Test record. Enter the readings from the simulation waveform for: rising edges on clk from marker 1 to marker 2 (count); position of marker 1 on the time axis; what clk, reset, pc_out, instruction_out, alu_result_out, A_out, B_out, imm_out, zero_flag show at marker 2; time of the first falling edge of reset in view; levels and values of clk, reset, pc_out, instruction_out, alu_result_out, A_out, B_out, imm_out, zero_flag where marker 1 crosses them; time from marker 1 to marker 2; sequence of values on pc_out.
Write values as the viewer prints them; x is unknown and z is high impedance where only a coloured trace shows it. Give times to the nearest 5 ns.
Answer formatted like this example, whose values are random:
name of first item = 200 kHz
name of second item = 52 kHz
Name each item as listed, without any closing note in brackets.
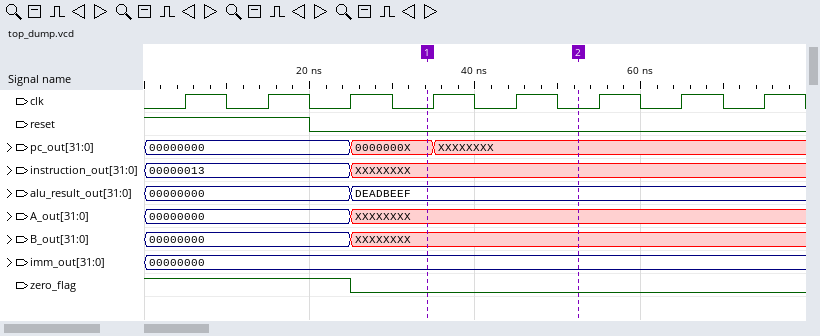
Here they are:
rising edges on clk from marker 1 to marker 2 = 2
position of marker 1 on the time axis = 35 ns
what clk, reset, pc_out, instruction_out, alu_result_out, A_out, B_out, imm_out, zero_flag show at marker 2 = clk=0, reset=0, pc_out=XXXXXXXX, instruction_out=XXXXXXXX, alu_result_out=DEADBEEF, A_out=XXXXXXXX, B_out=XXXXXXXX, imm_out=00000000, zero_flag=0
time of the first falling edge of reset in view = 20 ns
levels and values of clk, reset, pc_out, instruction_out, alu_result_out, A_out, B_out, imm_out, zero_flag where marker 1 crosses them = clk=0, reset=0, pc_out=0000000X, instruction_out=XXXXXXXX, alu_result_out=DEADBEEF, A_out=XXXXXXXX, B_out=XXXXXXXX, imm_out=00000000, zero_flag=0
time from marker 1 to marker 2 = 20 ns
sequence of values on pc_out = 00000000, 0000000X, XXXXXXXX
